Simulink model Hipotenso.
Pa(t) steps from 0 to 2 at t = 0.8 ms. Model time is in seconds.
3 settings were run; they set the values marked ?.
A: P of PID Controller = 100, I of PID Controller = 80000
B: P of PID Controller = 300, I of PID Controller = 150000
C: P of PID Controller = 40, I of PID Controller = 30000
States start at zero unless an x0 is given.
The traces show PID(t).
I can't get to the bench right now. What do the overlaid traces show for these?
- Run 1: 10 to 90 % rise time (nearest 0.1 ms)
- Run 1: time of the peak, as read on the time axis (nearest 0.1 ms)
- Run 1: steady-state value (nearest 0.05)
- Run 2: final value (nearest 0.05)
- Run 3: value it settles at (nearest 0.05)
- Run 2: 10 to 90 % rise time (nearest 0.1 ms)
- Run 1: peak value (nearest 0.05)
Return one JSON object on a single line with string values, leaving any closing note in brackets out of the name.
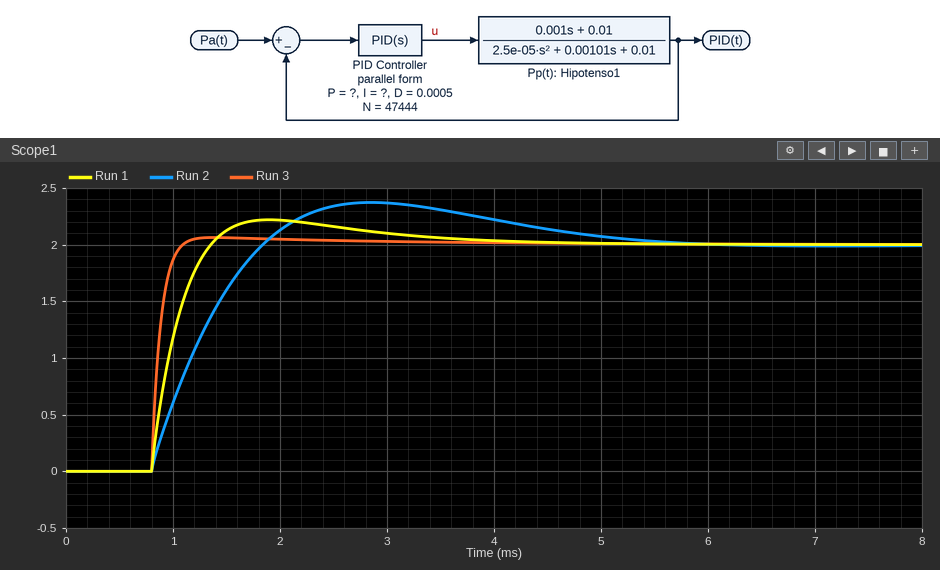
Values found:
{"Run 1: 10 to 90 % rise time": "0.4 ms", "Run 1: time of the peak, as read on the time axis": "1.9 ms", "Run 1: steady-state value": "2.00", "Run 2: final value": "2.00", "Run 3: value it settles at": "2.00", "Run 2: 10 to 90 % rise time": "0.8 ms", "Run 1: peak value": "2.20"}
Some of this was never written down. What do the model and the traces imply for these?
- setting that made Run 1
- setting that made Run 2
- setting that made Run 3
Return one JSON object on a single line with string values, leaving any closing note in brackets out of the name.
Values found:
{"setting that made Run 1": "A", "setting that made Run 2": "C", "setting that made Run 3": "B"}
